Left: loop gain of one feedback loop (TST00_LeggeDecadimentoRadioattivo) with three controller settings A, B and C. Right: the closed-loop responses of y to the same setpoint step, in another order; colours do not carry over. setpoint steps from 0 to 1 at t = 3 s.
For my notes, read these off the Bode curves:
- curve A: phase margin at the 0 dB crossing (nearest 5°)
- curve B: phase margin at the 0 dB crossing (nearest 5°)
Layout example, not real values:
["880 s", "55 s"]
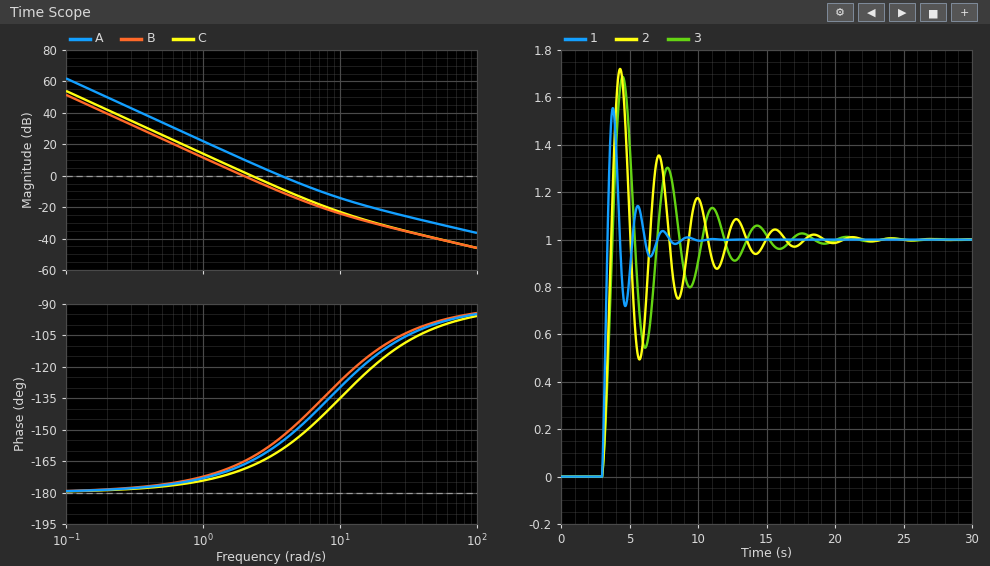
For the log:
["25°", "15°"]
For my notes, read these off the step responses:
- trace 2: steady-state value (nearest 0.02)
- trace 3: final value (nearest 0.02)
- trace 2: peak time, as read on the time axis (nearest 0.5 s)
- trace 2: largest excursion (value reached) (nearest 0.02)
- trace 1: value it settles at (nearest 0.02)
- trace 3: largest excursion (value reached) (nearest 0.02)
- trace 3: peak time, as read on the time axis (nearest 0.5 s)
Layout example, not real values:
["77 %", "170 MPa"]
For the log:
["1.00", "1.00", "4.5 s", "1.72", "1.00", "1.68", "4.5 s"]
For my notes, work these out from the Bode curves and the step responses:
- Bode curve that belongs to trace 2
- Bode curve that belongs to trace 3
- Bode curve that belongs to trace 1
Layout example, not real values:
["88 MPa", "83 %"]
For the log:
["C", "B", "A"]
